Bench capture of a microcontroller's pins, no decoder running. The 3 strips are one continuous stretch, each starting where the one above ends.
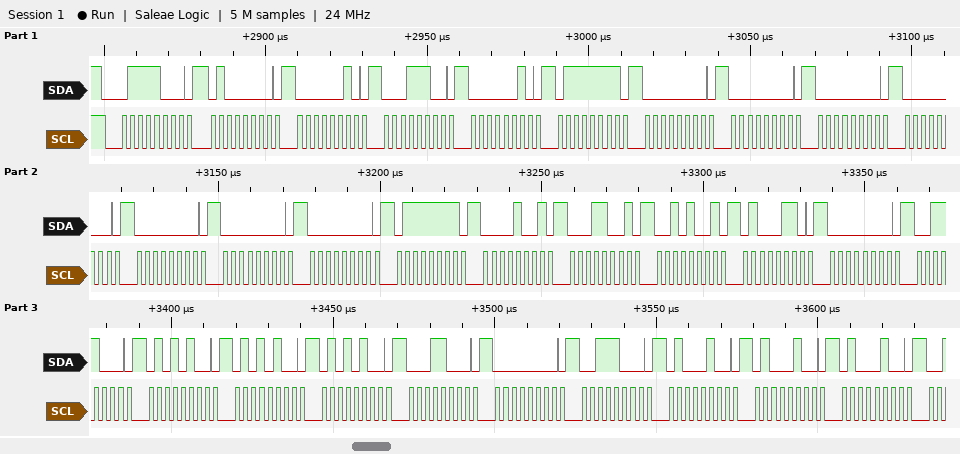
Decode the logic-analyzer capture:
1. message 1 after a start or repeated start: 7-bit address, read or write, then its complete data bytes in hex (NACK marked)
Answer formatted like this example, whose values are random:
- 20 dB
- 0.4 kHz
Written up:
- 0x3C write: 40 02 1C 02 7F 00 00 00 00 00 00 00 7F 09 19 29 46 00 38 54 54 54 18 00 38 44 44 44
